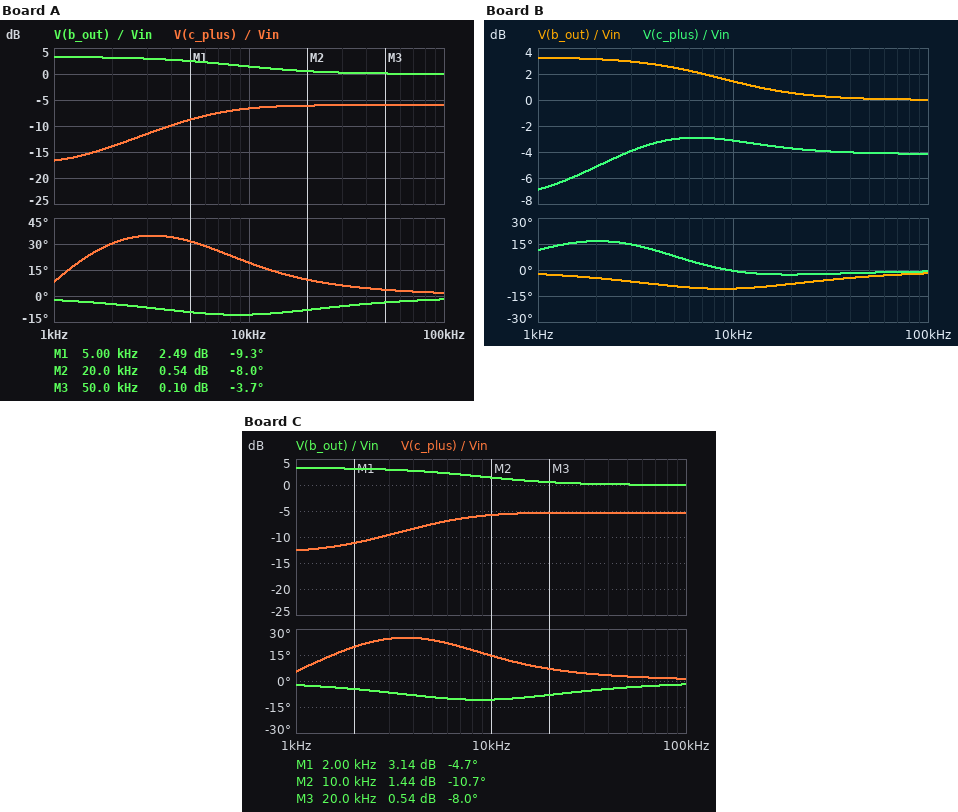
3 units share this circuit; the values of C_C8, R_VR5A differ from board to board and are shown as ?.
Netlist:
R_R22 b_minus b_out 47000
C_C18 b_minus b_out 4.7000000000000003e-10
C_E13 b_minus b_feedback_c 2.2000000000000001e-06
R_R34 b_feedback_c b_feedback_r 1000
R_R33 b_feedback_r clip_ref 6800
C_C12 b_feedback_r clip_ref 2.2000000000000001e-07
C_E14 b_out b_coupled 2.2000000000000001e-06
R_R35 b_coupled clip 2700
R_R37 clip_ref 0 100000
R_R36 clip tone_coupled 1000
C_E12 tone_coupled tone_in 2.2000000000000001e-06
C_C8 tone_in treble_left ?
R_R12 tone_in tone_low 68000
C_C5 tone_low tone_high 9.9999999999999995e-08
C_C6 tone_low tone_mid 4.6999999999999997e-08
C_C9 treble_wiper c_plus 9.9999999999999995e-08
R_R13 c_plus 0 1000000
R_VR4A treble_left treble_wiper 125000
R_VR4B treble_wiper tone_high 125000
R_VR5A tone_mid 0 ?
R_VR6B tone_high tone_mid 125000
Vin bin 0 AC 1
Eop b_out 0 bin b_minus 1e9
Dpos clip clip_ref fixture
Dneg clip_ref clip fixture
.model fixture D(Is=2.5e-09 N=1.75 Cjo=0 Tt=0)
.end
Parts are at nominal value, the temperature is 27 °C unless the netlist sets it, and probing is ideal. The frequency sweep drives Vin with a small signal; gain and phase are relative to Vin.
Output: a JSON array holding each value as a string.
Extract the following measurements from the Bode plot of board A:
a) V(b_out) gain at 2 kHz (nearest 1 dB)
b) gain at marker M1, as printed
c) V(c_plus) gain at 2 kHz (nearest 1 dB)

["3 dB", "2.49 dB", "-14 dB"]
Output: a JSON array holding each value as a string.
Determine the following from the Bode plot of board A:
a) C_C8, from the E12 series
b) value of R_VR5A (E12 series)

["82 pF", "8.2 kΩ"]
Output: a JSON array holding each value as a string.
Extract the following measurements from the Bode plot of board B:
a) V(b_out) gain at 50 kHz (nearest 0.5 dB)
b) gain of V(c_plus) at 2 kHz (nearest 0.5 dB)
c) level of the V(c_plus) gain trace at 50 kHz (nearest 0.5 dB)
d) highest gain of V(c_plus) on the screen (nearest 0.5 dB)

["0 dB", "-5.0 dB", "-4.0 dB", "-3.0 dB"]
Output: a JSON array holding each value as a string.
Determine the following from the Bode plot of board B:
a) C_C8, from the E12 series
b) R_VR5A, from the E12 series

["180 pF", "33 kΩ"]
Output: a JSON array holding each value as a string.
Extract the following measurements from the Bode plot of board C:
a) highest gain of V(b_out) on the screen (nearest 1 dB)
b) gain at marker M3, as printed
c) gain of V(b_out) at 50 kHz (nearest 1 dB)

["3 dB", "0.54 dB", "0 dB"]
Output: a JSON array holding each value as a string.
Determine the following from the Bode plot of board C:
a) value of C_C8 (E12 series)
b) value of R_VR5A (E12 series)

["82 pF", "15 kΩ"]
